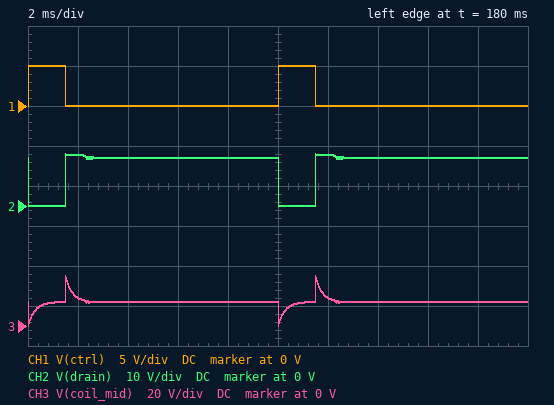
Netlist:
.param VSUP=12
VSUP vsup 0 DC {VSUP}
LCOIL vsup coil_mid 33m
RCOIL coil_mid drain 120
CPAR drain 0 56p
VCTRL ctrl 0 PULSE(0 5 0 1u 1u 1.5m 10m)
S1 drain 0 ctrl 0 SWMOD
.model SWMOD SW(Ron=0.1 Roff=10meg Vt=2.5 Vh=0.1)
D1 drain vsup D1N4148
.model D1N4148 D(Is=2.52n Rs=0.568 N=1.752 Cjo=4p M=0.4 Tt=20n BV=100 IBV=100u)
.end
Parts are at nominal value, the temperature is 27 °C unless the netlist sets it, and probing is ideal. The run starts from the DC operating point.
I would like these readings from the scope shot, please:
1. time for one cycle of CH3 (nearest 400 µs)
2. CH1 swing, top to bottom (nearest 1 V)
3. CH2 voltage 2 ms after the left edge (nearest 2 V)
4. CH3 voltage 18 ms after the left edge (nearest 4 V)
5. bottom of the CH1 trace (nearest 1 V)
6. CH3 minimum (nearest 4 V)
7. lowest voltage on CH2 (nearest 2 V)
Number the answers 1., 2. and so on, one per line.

1. 10.0 ms
2. 5 V
3. 12 V
4. 12 V
5. 0 V
6. 0 V
7. 0 V
